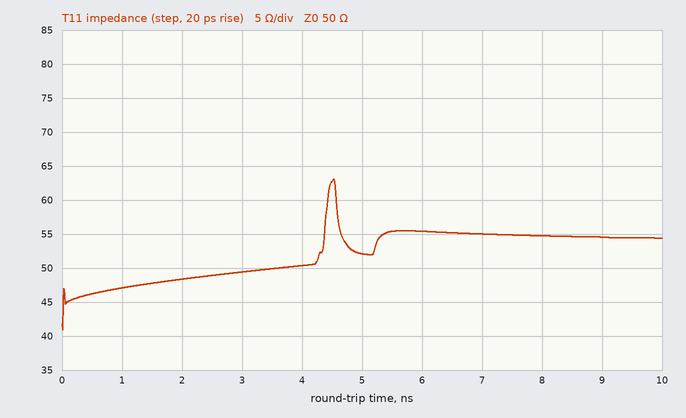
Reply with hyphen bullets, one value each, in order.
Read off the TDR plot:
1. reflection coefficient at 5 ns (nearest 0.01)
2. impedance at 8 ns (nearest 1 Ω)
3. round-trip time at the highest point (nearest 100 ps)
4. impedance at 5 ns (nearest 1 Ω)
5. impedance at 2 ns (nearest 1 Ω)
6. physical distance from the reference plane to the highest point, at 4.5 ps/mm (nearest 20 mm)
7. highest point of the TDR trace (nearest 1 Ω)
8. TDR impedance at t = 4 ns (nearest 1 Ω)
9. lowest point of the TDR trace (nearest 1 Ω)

- +0.02
- 55 Ω
- 4.5 ns
- 52 Ω
- 48 Ω
- 500 mm
- 63 Ω
- 50 Ω
- 41 Ω
